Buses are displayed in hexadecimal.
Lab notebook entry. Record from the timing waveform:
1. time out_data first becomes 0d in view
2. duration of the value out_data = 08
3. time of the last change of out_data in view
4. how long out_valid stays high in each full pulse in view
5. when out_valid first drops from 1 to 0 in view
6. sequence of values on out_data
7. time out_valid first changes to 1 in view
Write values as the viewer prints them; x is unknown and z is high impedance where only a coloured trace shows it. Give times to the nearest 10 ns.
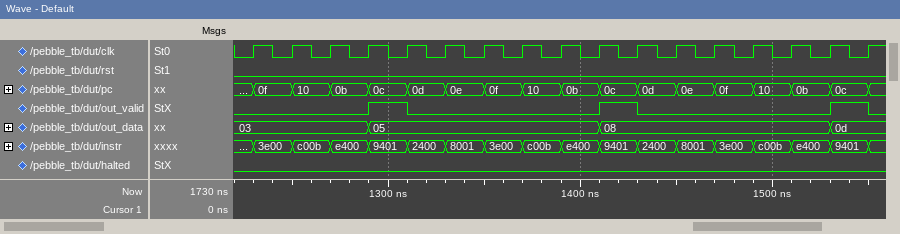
1530 ns
120 ns
1530 ns
20 ns, 20 ns, 20 ns
1310 ns
03, 05, 08, 0d
1290 ns
